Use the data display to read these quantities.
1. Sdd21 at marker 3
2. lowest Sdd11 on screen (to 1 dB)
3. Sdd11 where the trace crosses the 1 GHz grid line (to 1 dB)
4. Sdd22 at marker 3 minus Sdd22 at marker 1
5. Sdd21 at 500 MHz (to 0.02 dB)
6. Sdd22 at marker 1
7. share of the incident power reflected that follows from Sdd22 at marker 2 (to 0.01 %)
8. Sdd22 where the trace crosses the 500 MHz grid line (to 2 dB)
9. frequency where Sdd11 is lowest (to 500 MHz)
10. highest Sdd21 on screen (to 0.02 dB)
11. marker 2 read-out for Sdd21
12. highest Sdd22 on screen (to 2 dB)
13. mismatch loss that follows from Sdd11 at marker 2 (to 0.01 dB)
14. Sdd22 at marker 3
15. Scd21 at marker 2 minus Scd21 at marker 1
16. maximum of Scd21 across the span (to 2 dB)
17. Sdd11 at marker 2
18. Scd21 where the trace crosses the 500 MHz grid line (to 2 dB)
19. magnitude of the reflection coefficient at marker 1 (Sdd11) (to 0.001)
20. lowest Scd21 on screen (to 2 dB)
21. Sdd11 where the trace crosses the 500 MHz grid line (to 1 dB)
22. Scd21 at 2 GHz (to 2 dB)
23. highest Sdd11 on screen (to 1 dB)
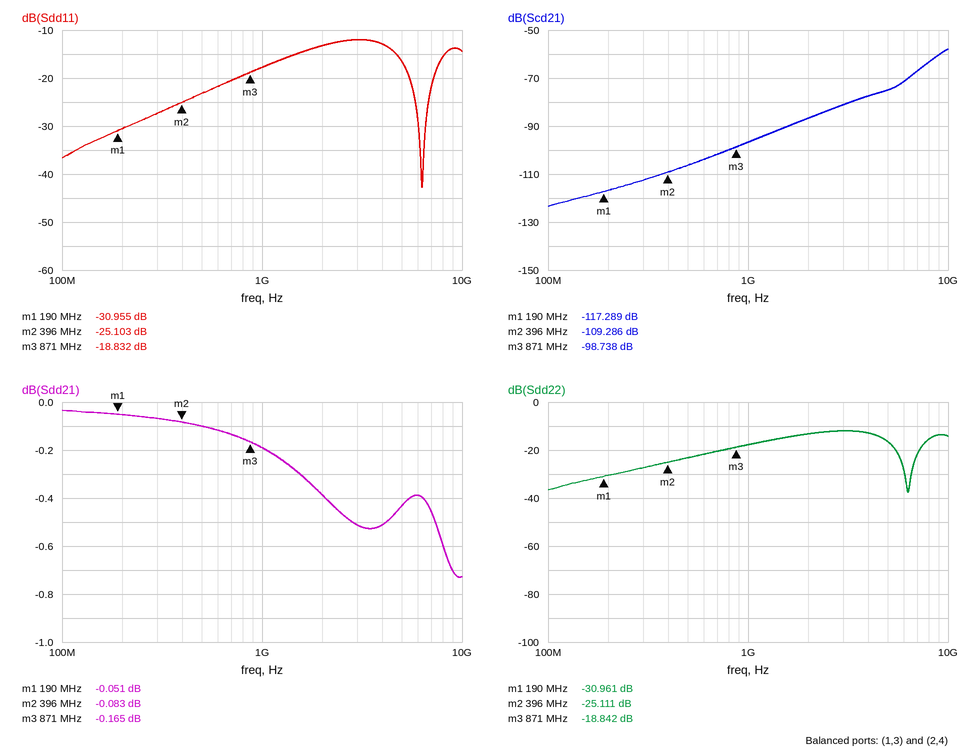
-0.165 dB
-43 dB
-18 dB
12.119 dB
-0.10 dB
-30.961 dB
0.31 %
-24 dB
6.5 GHz
-0.04 dB
-0.083 dB
-12 dB
0.01 dB
-18.842 dB
8.003 dB
-58 dB
-25.103 dB
-106 dB
0.028
-124 dB
-23 dB
-86 dB
-12 dB
